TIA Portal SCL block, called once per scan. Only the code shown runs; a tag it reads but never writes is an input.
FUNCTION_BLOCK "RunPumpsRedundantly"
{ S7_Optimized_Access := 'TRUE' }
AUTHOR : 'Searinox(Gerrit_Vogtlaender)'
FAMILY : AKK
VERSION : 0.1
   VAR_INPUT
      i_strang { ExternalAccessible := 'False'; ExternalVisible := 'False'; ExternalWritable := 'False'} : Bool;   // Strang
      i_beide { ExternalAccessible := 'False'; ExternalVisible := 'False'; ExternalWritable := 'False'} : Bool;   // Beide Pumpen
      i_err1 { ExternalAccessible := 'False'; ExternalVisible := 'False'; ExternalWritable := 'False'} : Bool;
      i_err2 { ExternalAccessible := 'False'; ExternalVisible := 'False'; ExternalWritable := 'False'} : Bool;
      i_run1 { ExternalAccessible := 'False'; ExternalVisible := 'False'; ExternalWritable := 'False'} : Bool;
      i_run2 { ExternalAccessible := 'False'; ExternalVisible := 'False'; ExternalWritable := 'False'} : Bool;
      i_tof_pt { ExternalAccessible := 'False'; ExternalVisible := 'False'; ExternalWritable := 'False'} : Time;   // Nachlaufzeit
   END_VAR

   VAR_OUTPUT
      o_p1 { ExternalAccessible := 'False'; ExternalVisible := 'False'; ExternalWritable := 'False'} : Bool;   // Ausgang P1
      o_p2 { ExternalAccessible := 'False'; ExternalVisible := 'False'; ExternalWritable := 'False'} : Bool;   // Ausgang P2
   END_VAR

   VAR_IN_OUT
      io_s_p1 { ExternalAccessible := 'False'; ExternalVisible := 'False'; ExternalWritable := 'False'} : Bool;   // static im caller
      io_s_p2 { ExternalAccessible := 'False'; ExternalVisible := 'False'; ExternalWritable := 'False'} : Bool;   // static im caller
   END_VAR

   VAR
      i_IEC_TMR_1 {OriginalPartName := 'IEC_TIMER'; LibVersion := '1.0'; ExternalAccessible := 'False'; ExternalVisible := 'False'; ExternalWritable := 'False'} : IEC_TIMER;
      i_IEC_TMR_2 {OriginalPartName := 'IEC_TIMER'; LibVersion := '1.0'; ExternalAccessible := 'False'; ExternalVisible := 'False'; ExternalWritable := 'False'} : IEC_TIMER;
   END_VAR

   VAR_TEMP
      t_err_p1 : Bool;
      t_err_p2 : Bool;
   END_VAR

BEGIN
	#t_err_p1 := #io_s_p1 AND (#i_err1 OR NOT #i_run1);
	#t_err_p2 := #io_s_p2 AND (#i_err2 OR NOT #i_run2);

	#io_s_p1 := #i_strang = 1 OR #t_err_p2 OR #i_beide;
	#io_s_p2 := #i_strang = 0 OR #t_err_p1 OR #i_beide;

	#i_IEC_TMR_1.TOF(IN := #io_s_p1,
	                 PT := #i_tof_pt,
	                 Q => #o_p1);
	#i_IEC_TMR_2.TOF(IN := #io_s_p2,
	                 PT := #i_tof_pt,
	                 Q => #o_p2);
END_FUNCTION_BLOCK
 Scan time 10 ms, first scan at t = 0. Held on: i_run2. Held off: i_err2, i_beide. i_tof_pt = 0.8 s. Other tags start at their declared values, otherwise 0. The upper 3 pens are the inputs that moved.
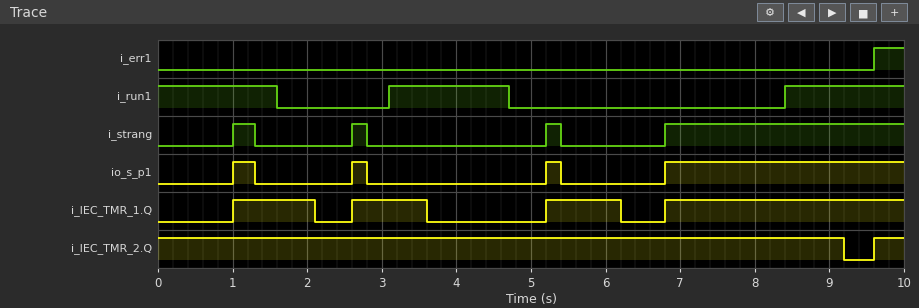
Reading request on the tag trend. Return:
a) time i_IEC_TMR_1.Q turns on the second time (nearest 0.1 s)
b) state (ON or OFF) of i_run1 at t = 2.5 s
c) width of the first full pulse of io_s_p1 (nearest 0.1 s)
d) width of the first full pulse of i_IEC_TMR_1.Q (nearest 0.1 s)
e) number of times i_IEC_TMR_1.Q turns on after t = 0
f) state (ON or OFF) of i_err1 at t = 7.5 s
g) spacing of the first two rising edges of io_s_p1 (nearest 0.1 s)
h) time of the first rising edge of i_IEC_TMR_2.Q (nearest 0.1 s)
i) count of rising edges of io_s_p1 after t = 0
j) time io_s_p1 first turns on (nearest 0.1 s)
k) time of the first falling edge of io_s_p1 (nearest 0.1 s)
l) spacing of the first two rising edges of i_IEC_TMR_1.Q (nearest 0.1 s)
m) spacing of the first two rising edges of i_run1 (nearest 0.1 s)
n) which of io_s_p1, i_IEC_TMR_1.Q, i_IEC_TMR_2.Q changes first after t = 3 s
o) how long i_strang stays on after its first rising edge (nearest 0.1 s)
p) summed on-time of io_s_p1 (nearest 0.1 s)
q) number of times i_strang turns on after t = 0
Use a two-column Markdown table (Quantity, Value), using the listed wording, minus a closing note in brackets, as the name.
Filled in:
| Quantity | Value |
|---|---|
| time i_IEC_TMR_1.Q turns on the second time | 2.6 s |
| state (ON or OFF) of i_run1 at t = 2.5 s | OFF |
| width of the first full pulse of io_s_p1 | 0.3 s |
| width of the first full pulse of i_IEC_TMR_1.Q | 1.1 s |
| number of times i_IEC_TMR_1.Q turns on after t = 0 | 4 |
| state (ON or OFF) of i_err1 at t = 7.5 s | OFF |
| spacing of the first two rising edges of io_s_p1 | 1.6 s |
| time of the first rising edge of i_IEC_TMR_2.Q | 9.6 s |
| count of rising edges of io_s_p1 after t = 0 | 4 |
| time io_s_p1 first turns on | 1.0 s |
| time of the first falling edge of io_s_p1 | 1.3 s |
| spacing of the first two rising edges of i_IEC_TMR_1.Q | 1.6 s |
| spacing of the first two rising edges of i_run1 | 5.3 s |
| which of io_s_p1, i_IEC_TMR_1.Q, i_IEC_TMR_2.Q changes first after t = 3 s | i_IEC_TMR_1.Q |
| how long i_strang stays on after its first rising edge | 0.3 s |
| summed on-time of io_s_p1 | 3.9 s |
| number of times i_strang turns on after t = 0 | 4 |
